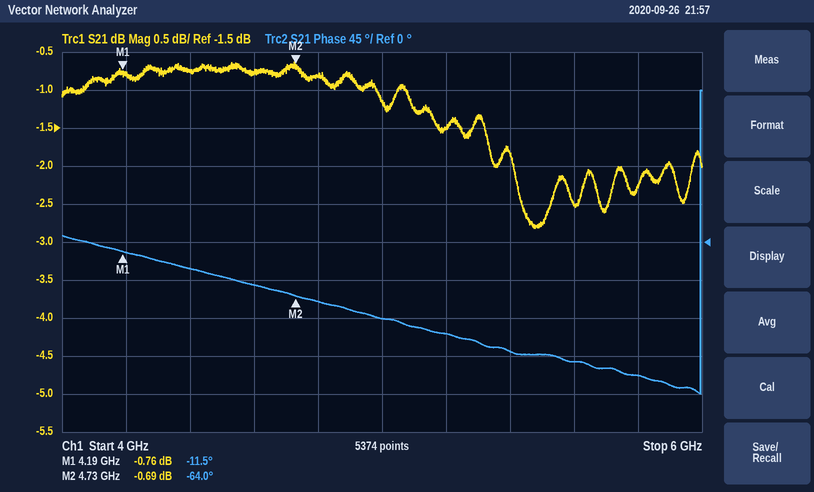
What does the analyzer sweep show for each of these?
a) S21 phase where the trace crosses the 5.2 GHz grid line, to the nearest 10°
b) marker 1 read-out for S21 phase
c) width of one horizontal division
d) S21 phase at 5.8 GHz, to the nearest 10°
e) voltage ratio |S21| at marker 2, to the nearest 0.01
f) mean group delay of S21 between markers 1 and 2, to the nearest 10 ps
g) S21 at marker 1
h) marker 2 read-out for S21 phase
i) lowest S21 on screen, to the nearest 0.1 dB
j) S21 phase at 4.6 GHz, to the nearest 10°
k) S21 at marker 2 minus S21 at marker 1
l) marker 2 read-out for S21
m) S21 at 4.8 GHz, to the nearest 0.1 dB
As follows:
-110°
-11.5°
200 MHz
-160°
0.92
270 ps
-0.76 dB
-64.0°
-2.8 dB
-50°
0.07 dB
-0.69 dB
-0.8 dB
